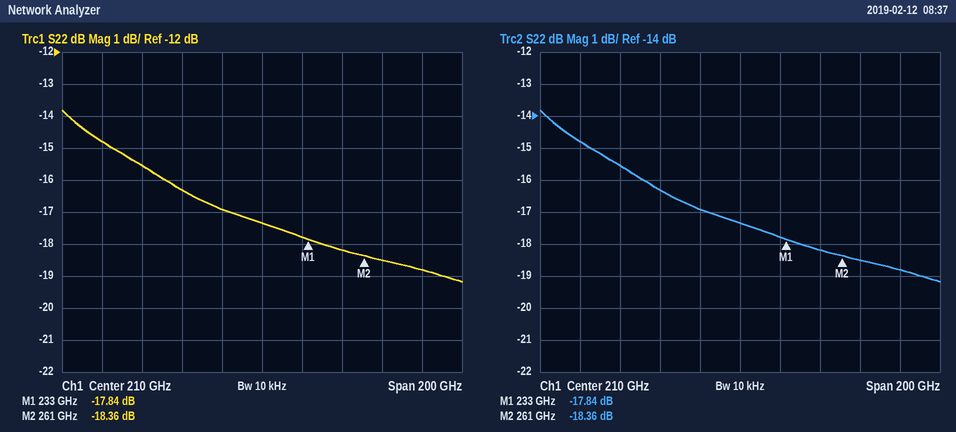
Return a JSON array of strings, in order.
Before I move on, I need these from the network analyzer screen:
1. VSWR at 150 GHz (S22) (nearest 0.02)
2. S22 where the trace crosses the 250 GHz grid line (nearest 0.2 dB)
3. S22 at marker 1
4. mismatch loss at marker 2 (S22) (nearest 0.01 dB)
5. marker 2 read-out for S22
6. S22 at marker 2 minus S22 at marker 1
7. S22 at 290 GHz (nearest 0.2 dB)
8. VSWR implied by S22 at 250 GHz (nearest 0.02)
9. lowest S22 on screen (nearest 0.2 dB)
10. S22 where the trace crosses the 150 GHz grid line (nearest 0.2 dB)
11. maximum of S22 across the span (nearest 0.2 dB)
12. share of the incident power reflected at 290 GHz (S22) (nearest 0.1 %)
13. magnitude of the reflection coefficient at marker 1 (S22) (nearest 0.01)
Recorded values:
["1.40", "-18.2 dB", "-17.84 dB", "0.06 dB", "-18.36 dB", "-0.52 dB", "-18.8 dB", "1.28", "-19.2 dB", "-15.6 dB", "-13.8 dB", "1.3 %", "0.13"]
